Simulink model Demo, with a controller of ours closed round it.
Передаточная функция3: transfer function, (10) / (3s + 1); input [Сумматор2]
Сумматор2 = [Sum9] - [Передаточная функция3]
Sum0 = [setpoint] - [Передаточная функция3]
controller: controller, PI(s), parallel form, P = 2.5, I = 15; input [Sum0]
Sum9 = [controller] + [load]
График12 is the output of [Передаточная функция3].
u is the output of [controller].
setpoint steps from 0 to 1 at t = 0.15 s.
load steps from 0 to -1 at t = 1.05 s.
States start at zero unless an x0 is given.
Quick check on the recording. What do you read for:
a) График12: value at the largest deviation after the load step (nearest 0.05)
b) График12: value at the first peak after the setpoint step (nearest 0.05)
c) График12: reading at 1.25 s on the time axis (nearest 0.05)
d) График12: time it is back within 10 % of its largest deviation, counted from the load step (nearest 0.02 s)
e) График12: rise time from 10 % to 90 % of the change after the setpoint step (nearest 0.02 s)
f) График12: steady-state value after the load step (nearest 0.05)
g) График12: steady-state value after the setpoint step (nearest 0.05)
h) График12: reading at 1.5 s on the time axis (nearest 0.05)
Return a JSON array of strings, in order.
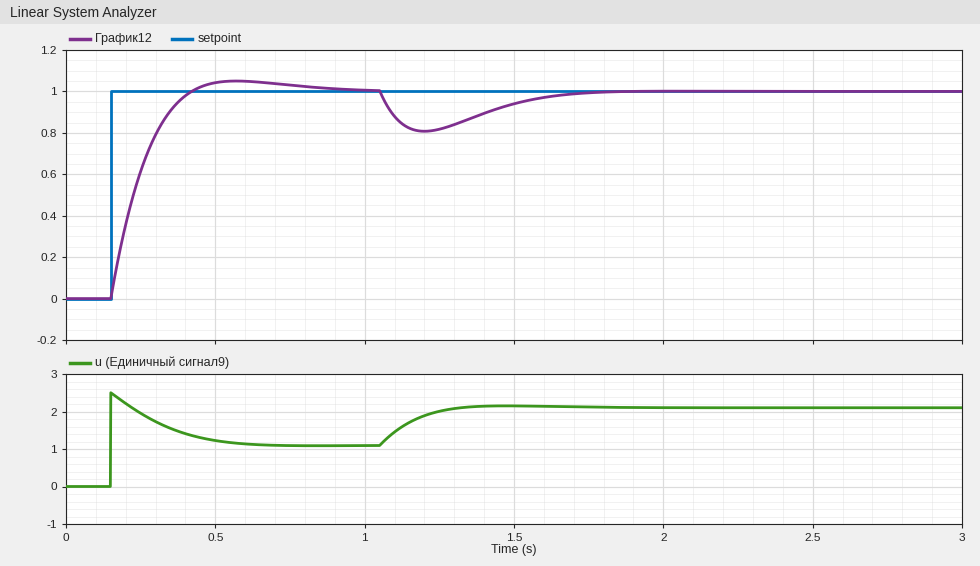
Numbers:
["0.80", "1.05", "0.80", "0.60 s", "0.18 s", "1.00", "1.00", "0.95"]
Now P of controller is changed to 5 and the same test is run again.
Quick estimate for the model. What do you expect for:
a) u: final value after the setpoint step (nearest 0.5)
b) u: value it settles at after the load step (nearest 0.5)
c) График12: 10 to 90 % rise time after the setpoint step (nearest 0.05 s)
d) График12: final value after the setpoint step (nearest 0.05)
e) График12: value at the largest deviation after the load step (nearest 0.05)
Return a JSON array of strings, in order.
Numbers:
["1.0", "2.0", "0.15 s", "1.00", "0.85"]
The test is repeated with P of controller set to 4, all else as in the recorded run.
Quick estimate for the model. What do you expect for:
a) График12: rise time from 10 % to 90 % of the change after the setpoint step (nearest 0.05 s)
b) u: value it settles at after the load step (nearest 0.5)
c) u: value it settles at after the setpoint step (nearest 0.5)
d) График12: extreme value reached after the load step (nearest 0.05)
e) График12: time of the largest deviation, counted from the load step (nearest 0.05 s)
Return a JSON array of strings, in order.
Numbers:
["0.15 s", "2.0", "1.0", "0.85", "0.15 s"]
